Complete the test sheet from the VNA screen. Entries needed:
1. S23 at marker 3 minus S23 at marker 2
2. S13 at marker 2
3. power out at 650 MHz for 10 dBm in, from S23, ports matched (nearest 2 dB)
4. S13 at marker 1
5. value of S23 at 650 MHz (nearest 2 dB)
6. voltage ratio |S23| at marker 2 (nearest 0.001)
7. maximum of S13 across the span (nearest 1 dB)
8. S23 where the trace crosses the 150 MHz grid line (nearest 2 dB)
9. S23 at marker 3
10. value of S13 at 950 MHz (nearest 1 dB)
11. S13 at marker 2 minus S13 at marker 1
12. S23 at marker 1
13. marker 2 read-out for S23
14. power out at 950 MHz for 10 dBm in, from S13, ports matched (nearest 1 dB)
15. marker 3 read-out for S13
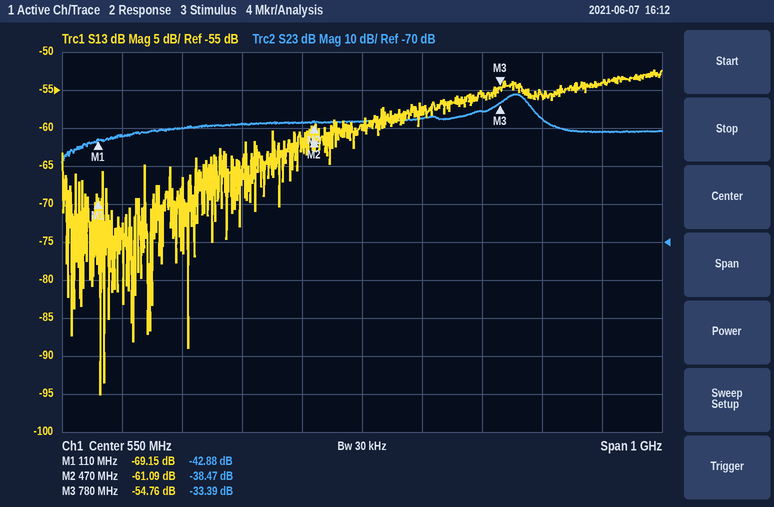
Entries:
5.08 dB
-61.09 dB
-28 dBm
-69.15 dB
-38 dB
0.012
-52 dB
-42 dB
-33.39 dB
-54 dB
8.06 dB
-42.88 dB
-38.47 dB
-44 dBm
-54.76 dB
